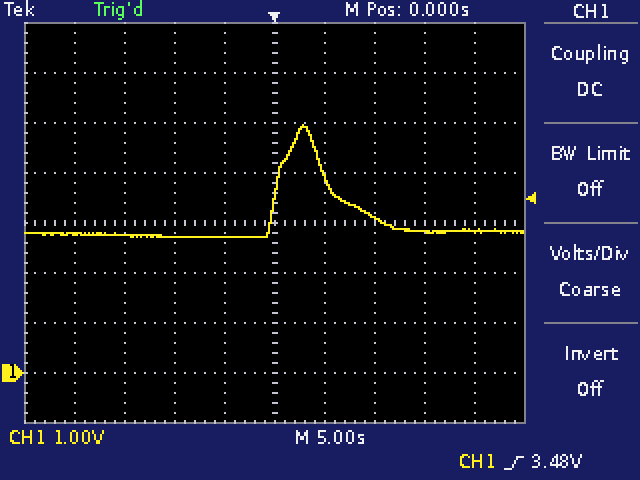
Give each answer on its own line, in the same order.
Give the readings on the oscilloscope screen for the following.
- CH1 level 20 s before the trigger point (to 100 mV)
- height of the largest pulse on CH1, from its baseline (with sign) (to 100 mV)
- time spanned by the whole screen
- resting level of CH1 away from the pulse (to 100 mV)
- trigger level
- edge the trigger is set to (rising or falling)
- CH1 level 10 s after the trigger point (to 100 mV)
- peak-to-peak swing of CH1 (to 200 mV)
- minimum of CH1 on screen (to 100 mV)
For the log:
2.8 V
+2.2 V
50 s
2.8 V
3.48 V
rising
3.1 V
2.2 V
2.7 V
